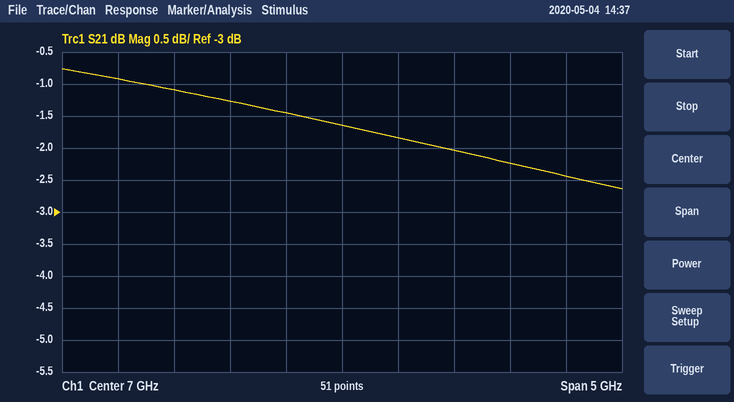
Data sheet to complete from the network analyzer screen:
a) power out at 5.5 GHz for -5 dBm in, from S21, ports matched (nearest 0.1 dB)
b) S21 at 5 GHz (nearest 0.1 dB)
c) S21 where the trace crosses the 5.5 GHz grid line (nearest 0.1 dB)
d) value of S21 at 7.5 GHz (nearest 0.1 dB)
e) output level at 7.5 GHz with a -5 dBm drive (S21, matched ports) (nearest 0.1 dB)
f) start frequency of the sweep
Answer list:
-6.1 dBm
-0.9 dB
-1.1 dB
-1.8 dB
-6.8 dBm
4.5 GHz
